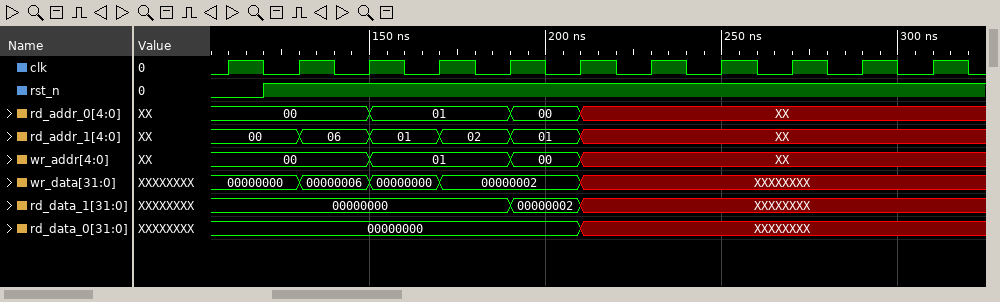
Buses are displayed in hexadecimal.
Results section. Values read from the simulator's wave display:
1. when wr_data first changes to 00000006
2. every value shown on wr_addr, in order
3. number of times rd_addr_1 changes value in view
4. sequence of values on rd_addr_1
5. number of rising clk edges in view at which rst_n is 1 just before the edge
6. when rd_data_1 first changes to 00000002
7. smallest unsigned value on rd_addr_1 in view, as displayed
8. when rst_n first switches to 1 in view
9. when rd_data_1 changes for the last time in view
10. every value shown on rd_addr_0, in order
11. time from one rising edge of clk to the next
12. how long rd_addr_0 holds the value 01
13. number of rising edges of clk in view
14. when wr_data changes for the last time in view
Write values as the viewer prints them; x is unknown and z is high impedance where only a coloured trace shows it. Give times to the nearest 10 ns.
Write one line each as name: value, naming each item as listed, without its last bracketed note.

when wr_data first changes to 00000006: 130 ns
every value shown on wr_addr, in order: 00, 01, 00, XX
number of times rd_addr_1 changes value in view: 5
sequence of values on rd_addr_1: 00, 06, 01, 02, 01, XX
number of rising clk edges in view at which rst_n is 1 just before the edge: 10
when rd_data_1 first changes to 00000002: 190 ns
smallest unsigned value on rd_addr_1 in view, as displayed: 00
when rst_n first switches to 1 in view: 120 ns
when rd_data_1 changes for the last time in view: 210 ns
every value shown on rd_addr_0, in order: 00, 01, 00, XX
time from one rising edge of clk to the next: 20 ns
how long rd_addr_0 holds the value 01: 40 ns
number of rising edges of clk in view: 11
when wr_data changes for the last time in view: 210 ns
